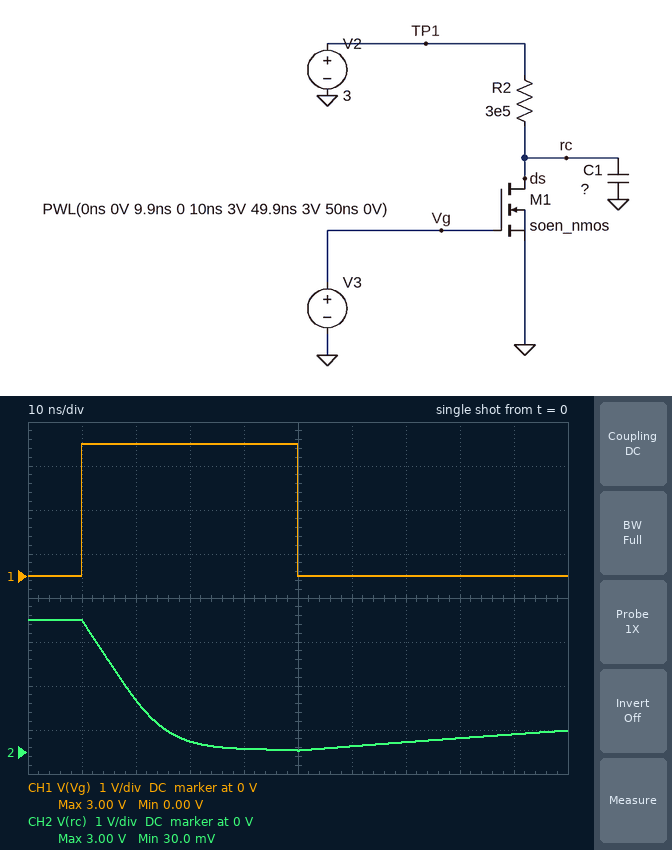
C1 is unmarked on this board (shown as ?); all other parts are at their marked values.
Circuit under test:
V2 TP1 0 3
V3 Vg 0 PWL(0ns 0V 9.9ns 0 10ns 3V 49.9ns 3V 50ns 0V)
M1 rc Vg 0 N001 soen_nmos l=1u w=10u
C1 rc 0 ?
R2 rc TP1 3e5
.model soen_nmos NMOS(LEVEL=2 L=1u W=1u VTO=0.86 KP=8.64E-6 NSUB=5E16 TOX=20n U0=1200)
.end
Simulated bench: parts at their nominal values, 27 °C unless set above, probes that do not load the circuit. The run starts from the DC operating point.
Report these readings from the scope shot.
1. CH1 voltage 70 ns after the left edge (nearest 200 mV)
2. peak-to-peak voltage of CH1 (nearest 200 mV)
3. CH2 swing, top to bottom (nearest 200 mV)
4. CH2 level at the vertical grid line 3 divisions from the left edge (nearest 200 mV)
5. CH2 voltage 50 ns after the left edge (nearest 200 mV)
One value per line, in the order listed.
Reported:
0 V
3.0 V
3.0 V
200 mV
0 V
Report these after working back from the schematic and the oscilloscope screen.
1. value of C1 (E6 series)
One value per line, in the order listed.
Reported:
1 pF
